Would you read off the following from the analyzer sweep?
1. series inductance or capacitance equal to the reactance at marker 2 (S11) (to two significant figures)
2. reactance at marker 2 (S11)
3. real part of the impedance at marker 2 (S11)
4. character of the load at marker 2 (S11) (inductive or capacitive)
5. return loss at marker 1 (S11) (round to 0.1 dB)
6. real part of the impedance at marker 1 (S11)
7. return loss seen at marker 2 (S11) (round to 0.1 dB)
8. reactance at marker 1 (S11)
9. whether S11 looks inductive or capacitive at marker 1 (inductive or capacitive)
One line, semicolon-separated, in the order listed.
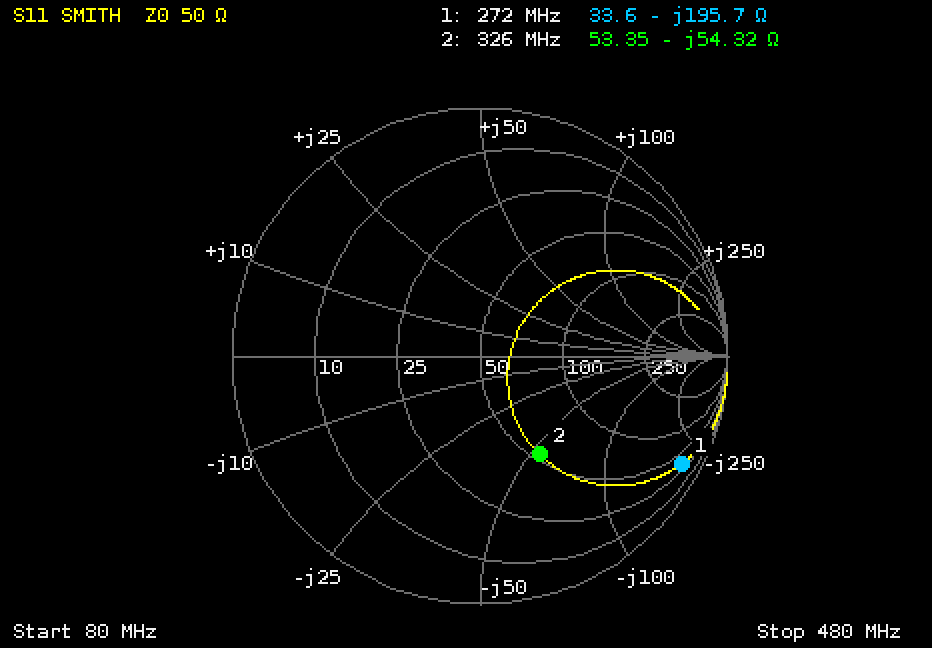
9.0 pF; -54.32 Ω; 53.35 Ω; capacitive; 0.7 dB; 33.6 Ω; 6.6 dB; -195.7 Ω; capacitive
